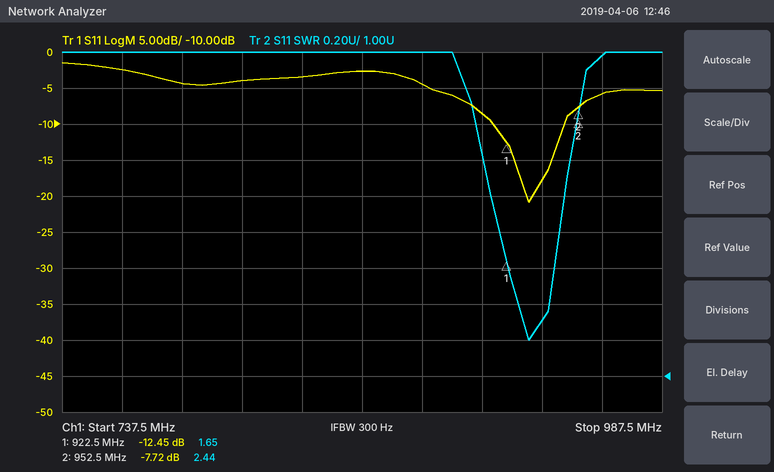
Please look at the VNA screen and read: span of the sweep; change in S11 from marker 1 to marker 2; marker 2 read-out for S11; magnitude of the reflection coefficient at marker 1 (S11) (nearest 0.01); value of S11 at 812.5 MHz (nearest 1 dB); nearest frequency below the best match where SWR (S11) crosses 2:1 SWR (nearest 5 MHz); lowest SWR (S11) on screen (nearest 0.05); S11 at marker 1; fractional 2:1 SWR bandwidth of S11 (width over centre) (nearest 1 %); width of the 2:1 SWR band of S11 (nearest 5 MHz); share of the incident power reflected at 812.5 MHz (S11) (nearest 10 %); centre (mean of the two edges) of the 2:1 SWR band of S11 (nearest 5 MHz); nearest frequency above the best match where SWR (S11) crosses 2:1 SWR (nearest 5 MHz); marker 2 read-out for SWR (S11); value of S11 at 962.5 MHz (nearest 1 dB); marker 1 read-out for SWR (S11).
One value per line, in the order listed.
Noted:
250 MHz
4.73 dB
-7.72 dB
0.24
-4 dB
915 MHz
1.20
-12.45 dB
3 %
30 MHz
40 %
930 MHz
945 MHz
2.44
-6 dB
1.65
